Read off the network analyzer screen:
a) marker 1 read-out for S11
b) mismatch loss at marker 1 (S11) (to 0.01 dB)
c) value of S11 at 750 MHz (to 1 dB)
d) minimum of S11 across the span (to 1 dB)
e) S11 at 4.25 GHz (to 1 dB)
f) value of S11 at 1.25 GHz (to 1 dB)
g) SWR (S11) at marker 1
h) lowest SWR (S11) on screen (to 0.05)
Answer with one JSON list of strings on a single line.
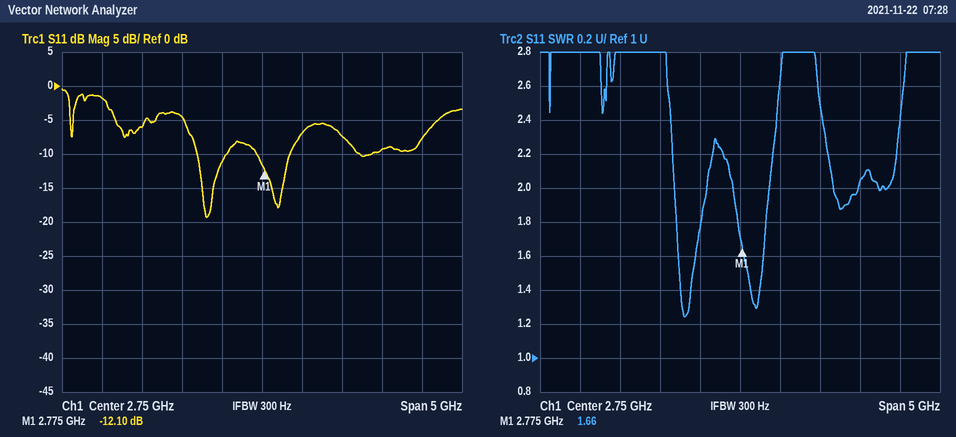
["-12.10 dB", "0.28 dB", "-2 dB", "-19 dB", "-9 dB", "-6 dB", "1.66", "1.25"]
